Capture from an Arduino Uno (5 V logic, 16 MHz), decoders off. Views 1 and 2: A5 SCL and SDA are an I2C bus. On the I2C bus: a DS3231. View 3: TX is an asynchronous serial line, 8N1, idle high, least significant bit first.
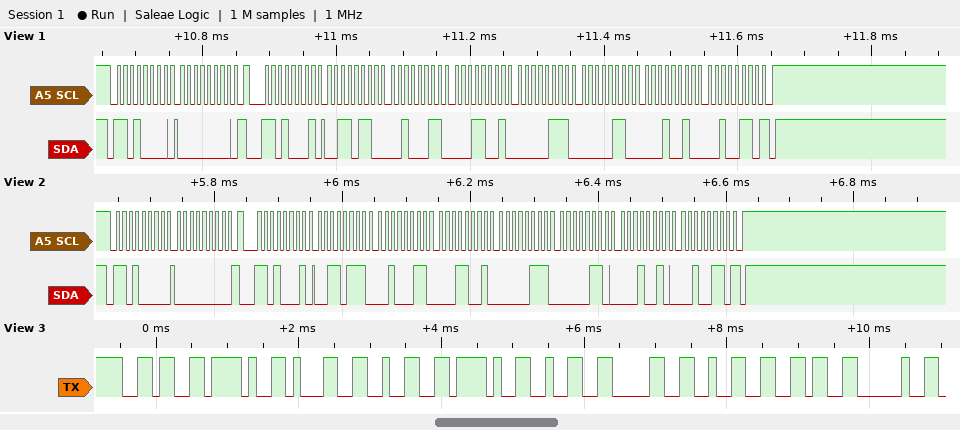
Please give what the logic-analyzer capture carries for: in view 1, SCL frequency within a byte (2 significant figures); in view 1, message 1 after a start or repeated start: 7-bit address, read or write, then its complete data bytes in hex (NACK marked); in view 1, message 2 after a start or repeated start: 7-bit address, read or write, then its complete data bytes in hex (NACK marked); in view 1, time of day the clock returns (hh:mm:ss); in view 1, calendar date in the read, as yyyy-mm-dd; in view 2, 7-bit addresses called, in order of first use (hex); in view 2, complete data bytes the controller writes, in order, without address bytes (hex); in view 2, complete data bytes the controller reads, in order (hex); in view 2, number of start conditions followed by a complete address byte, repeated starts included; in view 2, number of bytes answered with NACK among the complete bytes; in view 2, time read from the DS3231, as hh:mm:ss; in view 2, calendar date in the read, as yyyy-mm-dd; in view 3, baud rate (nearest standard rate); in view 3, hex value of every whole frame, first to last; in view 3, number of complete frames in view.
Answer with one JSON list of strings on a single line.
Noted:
["100 kHz", "0x68 write: 00", "0x68 read: 36 23 19 07 06 12 26 NACK", "19:23:36", "2026-12-06", "0x68", "00", "37 23 19 07 06 12 26", "2", "1", "19:23:37", "2026-12-06", "9600 baud", "0x36 0x2F 0x31 0x32 0x2F 0x32 0x30 0x32 0x36 0x20", "10"]
